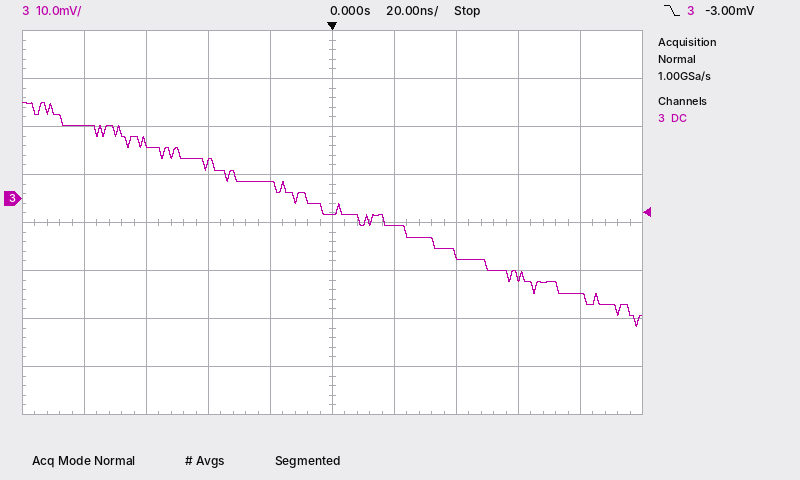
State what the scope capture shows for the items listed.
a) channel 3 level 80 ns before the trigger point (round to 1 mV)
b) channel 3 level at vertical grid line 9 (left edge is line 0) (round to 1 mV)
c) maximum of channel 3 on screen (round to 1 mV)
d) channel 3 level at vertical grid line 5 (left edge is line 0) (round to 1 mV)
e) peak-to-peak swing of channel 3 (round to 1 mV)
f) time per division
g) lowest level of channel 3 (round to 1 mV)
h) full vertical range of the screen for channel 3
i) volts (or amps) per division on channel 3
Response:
15 mV
-20 mV
20 mV
-3 mV
47 mV
20 ns
-27 mV
80 mV
10 mV
